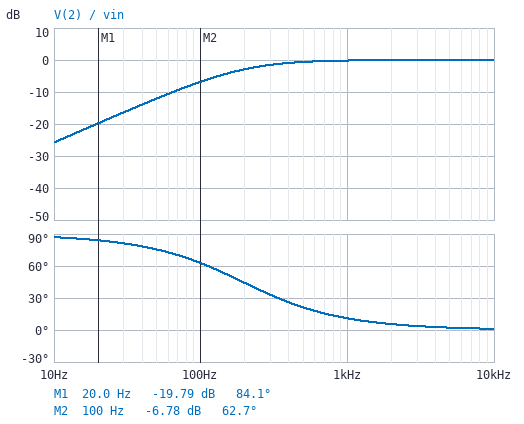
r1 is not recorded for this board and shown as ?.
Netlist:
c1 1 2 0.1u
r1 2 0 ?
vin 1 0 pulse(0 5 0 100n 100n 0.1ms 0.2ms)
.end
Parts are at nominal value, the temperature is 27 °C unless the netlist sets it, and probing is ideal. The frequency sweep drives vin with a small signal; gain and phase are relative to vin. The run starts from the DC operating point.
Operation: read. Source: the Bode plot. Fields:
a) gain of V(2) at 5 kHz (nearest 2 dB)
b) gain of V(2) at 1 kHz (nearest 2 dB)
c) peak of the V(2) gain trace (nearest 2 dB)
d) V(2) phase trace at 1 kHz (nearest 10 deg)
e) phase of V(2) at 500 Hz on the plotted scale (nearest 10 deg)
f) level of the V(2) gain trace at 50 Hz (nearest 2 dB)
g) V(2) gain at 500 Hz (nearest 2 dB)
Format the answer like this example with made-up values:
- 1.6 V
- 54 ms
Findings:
- 0 dB
- 0 dB
- 0 dB
- 10 deg
- 20 deg
- -12 dB
- 0 dB
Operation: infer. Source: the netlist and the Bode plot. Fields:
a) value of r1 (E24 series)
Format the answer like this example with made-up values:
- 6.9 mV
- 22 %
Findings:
- 8.2 kΩ
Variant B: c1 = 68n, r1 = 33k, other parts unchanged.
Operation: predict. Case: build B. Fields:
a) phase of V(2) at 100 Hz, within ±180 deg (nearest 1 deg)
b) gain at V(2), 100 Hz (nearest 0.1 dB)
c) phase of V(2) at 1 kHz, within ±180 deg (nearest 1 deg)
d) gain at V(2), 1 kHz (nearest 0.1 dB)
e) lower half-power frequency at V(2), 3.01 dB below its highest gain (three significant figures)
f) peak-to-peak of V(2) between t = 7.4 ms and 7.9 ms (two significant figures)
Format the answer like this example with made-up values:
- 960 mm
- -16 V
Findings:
- 35 deg
- -1.8 dB
- 4 deg
- 0 dB
- 70.9 Hz
- 5.1 V
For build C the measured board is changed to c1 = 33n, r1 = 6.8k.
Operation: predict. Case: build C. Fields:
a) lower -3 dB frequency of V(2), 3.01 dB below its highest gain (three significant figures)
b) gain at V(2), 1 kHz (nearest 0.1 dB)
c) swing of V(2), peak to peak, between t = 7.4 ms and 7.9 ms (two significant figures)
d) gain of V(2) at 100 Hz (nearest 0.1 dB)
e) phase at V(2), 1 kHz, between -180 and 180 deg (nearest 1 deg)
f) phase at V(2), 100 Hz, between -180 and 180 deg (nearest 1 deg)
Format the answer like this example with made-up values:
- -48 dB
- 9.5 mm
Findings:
- 709 Hz
- -1.8 dB
- 6.1 V
- -17.1 dB
- 35 deg
- 82 deg
